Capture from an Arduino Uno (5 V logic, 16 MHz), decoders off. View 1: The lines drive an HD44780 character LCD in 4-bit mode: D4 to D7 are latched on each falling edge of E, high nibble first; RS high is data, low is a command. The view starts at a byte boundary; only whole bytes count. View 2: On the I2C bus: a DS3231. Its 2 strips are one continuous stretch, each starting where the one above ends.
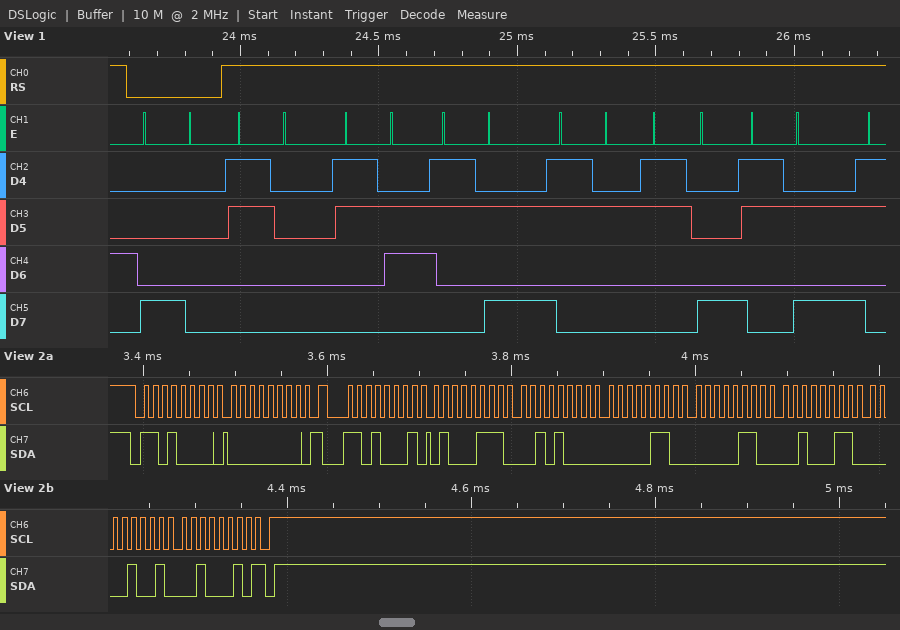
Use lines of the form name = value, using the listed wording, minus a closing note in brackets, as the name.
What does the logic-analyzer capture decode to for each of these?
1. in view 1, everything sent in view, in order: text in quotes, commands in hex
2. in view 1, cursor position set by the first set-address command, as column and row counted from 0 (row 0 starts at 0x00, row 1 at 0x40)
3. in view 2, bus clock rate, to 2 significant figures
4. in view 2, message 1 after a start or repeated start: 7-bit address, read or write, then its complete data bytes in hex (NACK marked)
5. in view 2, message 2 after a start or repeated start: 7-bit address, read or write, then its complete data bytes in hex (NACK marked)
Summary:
in view 1, everything sent in view, in order: text in quotes, commands in hex = 0x80 "06:28:"
in view 1, cursor position set by the first set-address command, as column and row counted from 0 = column 0, row 0
in view 2, bus clock rate, to 2 significant figures = 100 kHz
in view 2, message 1 after a start or repeated start: 7-bit address, read or write, then its complete data bytes in hex = 0x68 write: 00
in view 2, message 2 after a start or repeated start: 7-bit address, read or write, then its complete data bytes in hex = 0x68 read: 47 28 06 06 23 09 22 NACK
